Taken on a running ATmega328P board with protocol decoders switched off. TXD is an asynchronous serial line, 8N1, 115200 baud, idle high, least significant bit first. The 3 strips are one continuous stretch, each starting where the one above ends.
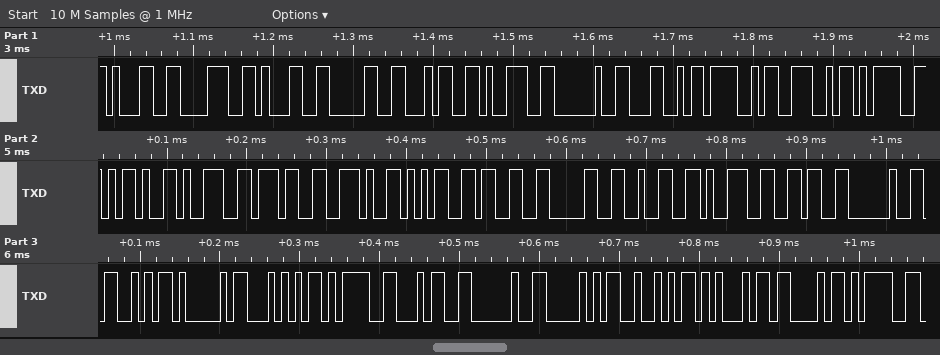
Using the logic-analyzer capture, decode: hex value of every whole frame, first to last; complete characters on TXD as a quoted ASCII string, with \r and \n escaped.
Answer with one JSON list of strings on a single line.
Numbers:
["31 38 31 30 34 39 20 4C 4F 4E 3D 2D 39 37 2E 35 33 30 32 39 36 20 53 41 54 3D 34 20 50 52 45 43 3D", "\"181049 LON=-97.530296 SAT=4 PREC=\""]
